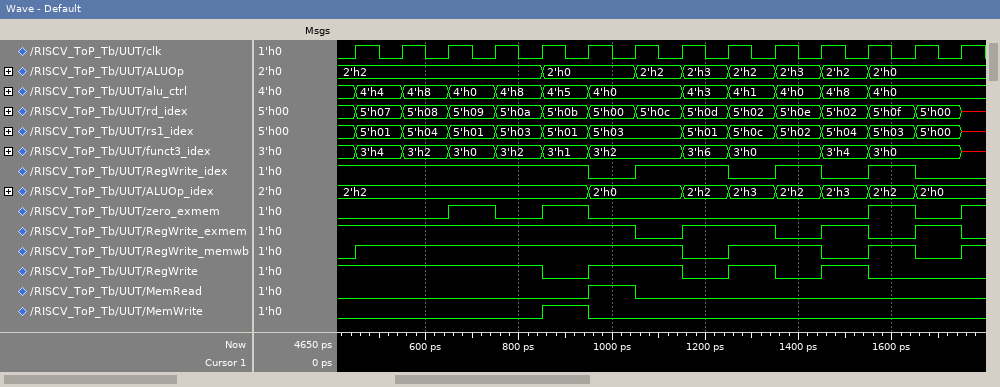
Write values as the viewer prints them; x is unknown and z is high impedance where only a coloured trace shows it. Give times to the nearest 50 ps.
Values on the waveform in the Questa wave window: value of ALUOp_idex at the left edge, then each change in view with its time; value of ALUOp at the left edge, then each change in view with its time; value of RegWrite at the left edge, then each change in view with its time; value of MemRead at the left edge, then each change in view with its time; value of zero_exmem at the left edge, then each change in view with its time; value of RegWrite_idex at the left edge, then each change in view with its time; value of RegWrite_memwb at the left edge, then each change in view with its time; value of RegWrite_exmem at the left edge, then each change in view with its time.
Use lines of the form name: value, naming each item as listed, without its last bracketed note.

value of ALUOp_idex at the left edge, then each change in view with its time: 2'h2, 2'h0 at 950 ps, 2'h2 at 1150 ps, 2'h3 at 1250 ps, 2'h2 at 1350 ps, 2'h3 at 1450 ps, 2'h2 at 1550 ps, 2'h0 at 1650 ps
value of ALUOp at the left edge, then each change in view with its time: 2'h2, 2'h0 at 850 ps, 2'h2 at 1050 ps, 2'h3 at 1150 ps, 2'h2 at 1250 ps, 2'h3 at 1350 ps, 2'h2 at 1450 ps, 2'h0 at 1550 ps
value of RegWrite at the left edge, then each change in view with its time: 1, 0 at 850 ps, 1 at 950 ps, 0 at 1150 ps, 1 at 1250 ps, 0 at 1350 ps, 1 at 1450 ps, 0 at 1550 ps
value of MemRead at the left edge, then each change in view with its time: 0, 1 at 950 ps, 0 at 1050 ps
value of zero_exmem at the left edge, then each change in view with its time: 0, 1 at 650 ps, 0 at 750 ps, 1 at 850 ps, 0 at 950 ps, 1 at 1550 ps, 0 at 1650 ps, 1 at 1750 ps
value of RegWrite_idex at the left edge, then each change in view with its time: 1, 0 at 950 ps, 1 at 1050 ps, 0 at 1250 ps, 1 at 1350 ps, 0 at 1450 ps, 1 at 1550 ps, 0 at 1650 ps
value of RegWrite_memwb at the left edge, then each change in view with its time: 0, 1 at 450 ps, 0 at 1150 ps, 1 at 1250 ps, 0 at 1450 ps, 1 at 1550 ps, 0 at 1650 ps, 1 at 1750 ps
value of RegWrite_exmem at the left edge, then each change in view with its time: 1, 0 at 1050 ps, 1 at 1150 ps, 0 at 1350 ps, 1 at 1450 ps, 0 at 1550 ps, 1 at 1650 ps, 0 at 1750 ps
